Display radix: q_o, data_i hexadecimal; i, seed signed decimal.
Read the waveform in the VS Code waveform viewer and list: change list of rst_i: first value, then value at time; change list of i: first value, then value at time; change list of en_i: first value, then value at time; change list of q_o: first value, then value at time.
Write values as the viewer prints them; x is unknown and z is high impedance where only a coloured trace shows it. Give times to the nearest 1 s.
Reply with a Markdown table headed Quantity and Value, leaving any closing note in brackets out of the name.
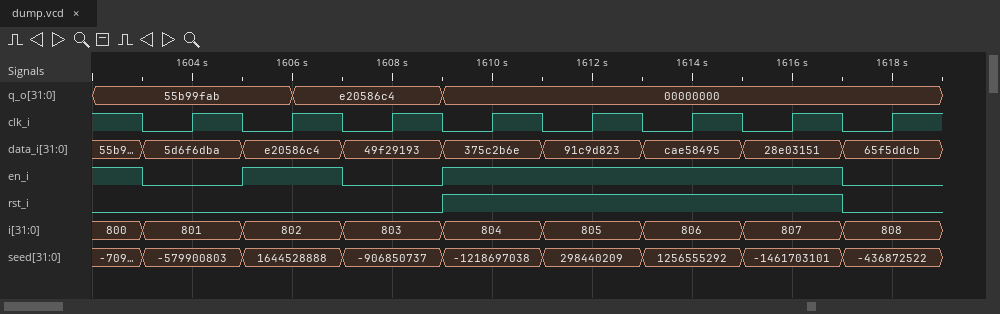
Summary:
| Quantity | Value |
|---|---|
| change list of rst_i: first value, then value at time | 0, 1 at 1609 s, 0 at 1617 s |
| change list of i: first value, then value at time | 800, 801 at 1603 s, 802 at 1605 s, 803 at 1607 s, 804 at 1609 s, 805 at 1611 s, 806 at 1613 s, 807 at 1615 s, 808 at 1617 s |
| change list of en_i: first value, then value at time | 1, 0 at 1603 s, 1 at 1605 s, 0 at 1607 s, 1 at 1609 s, 0 at 1617 s |
| change list of q_o: first value, then value at time | 55b99fab, e20586c4 at 1606 s, 00000000 at 1609 s |
